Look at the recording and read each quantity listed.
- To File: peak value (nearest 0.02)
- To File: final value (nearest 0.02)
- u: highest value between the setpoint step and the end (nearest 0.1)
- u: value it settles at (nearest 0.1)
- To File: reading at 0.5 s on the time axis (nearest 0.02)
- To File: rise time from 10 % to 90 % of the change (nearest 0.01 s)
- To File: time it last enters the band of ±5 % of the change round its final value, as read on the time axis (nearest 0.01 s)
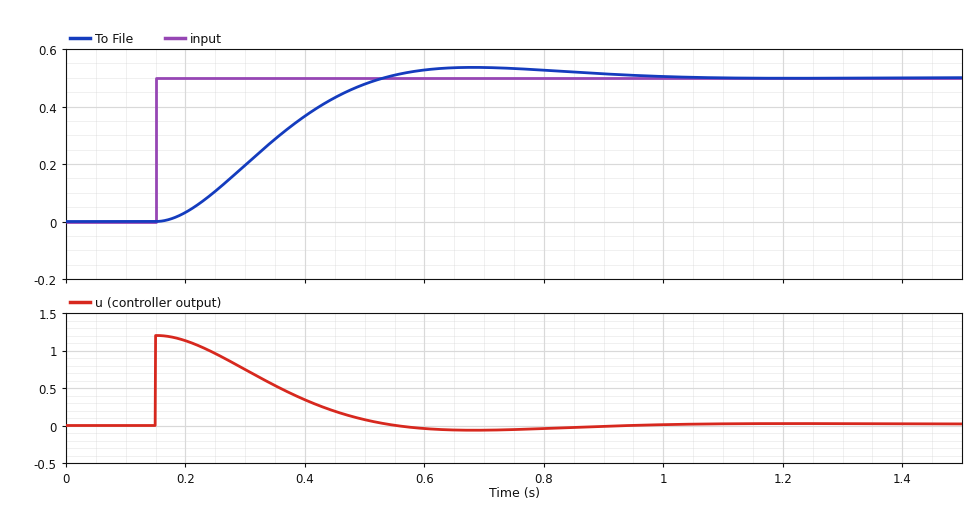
0.54
0.50
1.2
0.0
0.48
0.25 s
0.81 s
